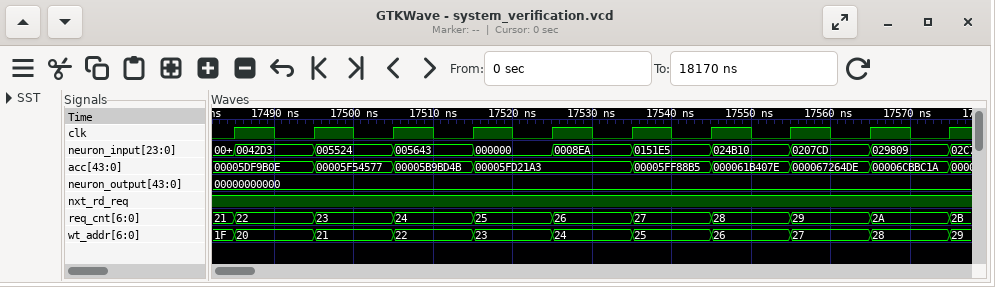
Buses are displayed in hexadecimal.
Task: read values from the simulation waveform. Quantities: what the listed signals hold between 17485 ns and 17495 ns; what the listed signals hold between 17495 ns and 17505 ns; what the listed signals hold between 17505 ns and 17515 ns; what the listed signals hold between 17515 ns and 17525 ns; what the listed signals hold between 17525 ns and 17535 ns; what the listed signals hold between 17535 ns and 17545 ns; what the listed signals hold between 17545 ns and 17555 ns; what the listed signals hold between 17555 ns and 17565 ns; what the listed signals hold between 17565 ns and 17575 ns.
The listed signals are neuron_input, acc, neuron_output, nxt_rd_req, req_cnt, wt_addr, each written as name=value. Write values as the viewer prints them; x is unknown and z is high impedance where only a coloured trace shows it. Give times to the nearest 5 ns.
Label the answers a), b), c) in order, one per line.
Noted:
a) neuron_input=0042D3, acc=00005DF9B0E, neuron_output=00000000000, nxt_rd_req=1, req_cnt=22, wt_addr=20
b) neuron_input=005524, acc=00005F54577, neuron_output=00000000000, nxt_rd_req=1, req_cnt=23, wt_addr=21
c) neuron_input=005643, acc=00005B9BD4B, neuron_output=00000000000, nxt_rd_req=1, req_cnt=24, wt_addr=22
d) neuron_input=000000, acc=00005FD21A3, neuron_output=00000000000, nxt_rd_req=1, req_cnt=25, wt_addr=23
e) neuron_input=0008EA, acc=00005FD21A3, neuron_output=00000000000, nxt_rd_req=1, req_cnt=26, wt_addr=24
f) neuron_input=0151E5, acc=00005FF88B5, neuron_output=00000000000, nxt_rd_req=1, req_cnt=27, wt_addr=25
g) neuron_input=024B10, acc=000061B407E, neuron_output=00000000000, nxt_rd_req=1, req_cnt=28, wt_addr=26
h) neuron_input=0207CD, acc=000067264DE, neuron_output=00000000000, nxt_rd_req=1, req_cnt=29, wt_addr=27
i) neuron_input=029809, acc=00006CBBC1A, neuron_output=00000000000, nxt_rd_req=1, req_cnt=2A, wt_addr=28
